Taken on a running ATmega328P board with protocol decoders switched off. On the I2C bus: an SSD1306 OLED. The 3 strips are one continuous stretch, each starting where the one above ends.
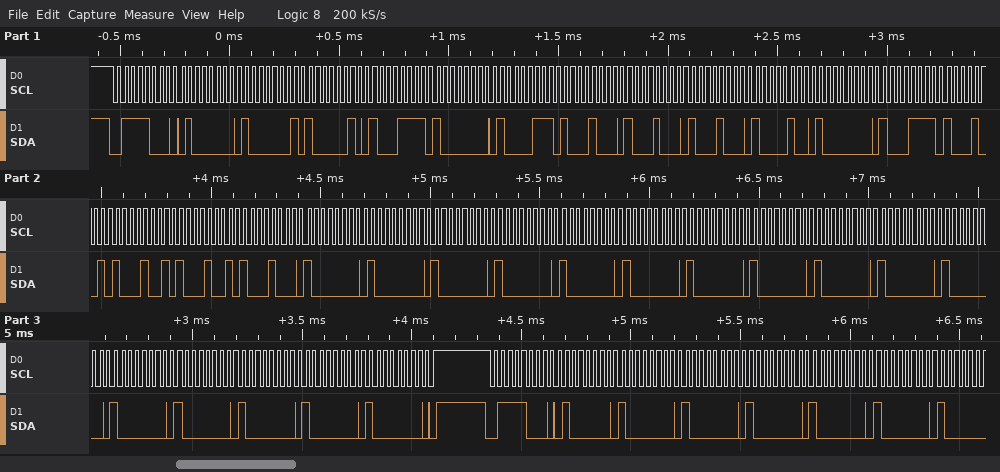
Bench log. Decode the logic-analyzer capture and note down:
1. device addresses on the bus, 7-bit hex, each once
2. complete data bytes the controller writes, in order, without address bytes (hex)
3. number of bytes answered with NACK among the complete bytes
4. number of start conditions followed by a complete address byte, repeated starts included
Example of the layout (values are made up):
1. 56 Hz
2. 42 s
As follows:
1. 0x3C
2. 40 81 82 8F 80 87 88 88 88 84 80 8F 89 89 89 88 80 80 80 80 80 80 80 80 80 80 80 80 80 80 80 80 40 80 80 80 80 80
3. 0
4. 2
